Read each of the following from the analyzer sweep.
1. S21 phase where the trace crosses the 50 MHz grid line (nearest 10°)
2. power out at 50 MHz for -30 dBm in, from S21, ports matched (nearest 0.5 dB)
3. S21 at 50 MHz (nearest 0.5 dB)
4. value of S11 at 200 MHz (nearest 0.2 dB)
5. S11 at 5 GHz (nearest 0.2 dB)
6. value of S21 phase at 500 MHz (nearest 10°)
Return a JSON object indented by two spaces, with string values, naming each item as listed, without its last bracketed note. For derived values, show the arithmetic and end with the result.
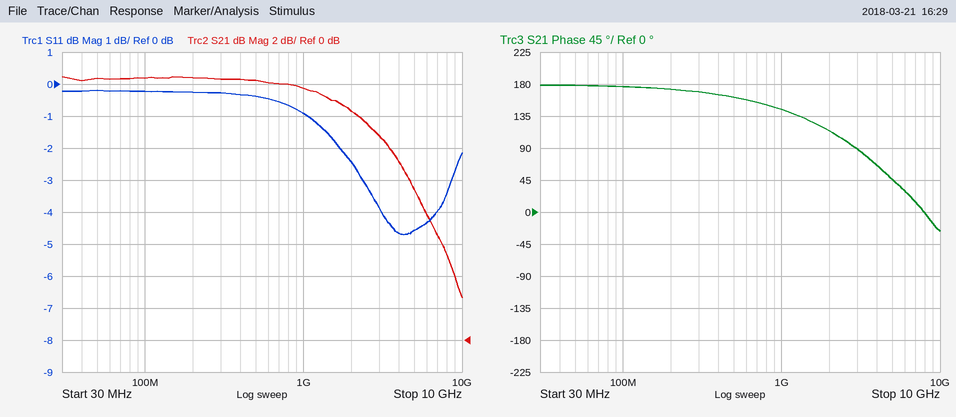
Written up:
{
  "S21 phase where the trace crosses the 50 MHz grid line": "180°",
  "power out at 50 MHz for -30 dBm in, from S21, ports matched": "-30 dBm + (16.5 dB) = -13.5 dBm",
  "S21 at 50 MHz": "16.5 dB",
  "value of S11 at 200 MHz": "-0.2 dB",
  "S11 at 5 GHz": "-4.6 dB",
  "value of S21 phase at 500 MHz": "160°"
}
